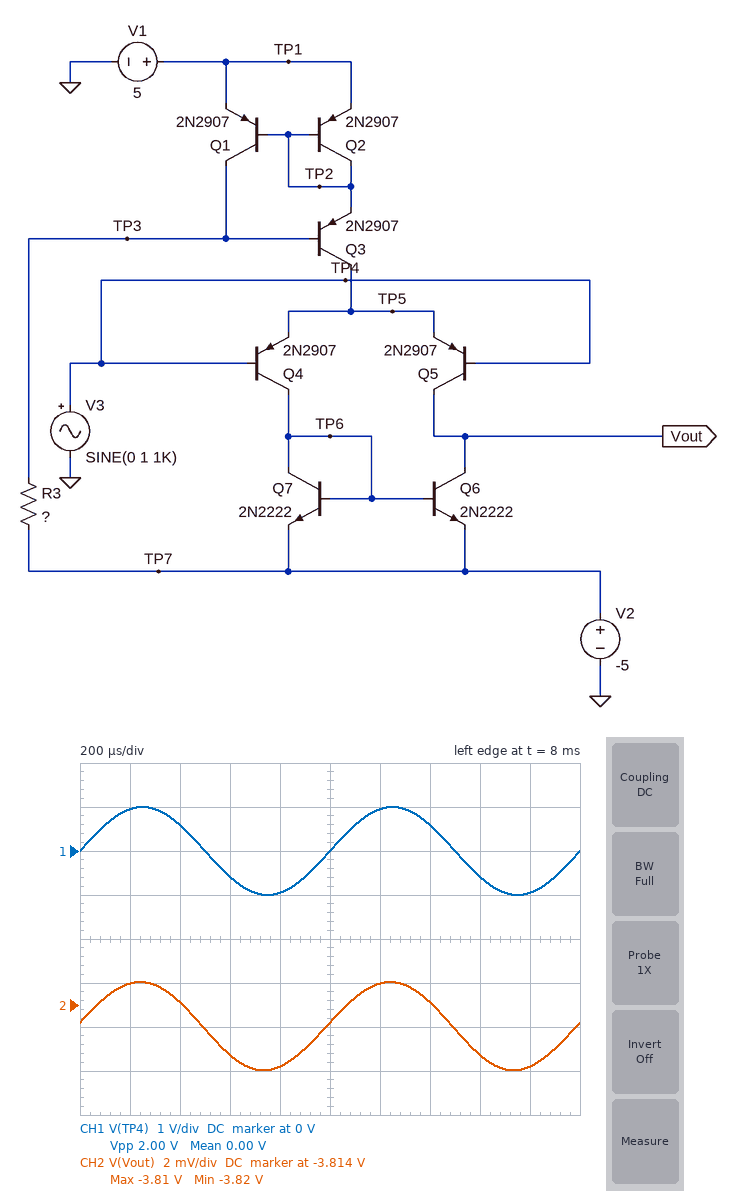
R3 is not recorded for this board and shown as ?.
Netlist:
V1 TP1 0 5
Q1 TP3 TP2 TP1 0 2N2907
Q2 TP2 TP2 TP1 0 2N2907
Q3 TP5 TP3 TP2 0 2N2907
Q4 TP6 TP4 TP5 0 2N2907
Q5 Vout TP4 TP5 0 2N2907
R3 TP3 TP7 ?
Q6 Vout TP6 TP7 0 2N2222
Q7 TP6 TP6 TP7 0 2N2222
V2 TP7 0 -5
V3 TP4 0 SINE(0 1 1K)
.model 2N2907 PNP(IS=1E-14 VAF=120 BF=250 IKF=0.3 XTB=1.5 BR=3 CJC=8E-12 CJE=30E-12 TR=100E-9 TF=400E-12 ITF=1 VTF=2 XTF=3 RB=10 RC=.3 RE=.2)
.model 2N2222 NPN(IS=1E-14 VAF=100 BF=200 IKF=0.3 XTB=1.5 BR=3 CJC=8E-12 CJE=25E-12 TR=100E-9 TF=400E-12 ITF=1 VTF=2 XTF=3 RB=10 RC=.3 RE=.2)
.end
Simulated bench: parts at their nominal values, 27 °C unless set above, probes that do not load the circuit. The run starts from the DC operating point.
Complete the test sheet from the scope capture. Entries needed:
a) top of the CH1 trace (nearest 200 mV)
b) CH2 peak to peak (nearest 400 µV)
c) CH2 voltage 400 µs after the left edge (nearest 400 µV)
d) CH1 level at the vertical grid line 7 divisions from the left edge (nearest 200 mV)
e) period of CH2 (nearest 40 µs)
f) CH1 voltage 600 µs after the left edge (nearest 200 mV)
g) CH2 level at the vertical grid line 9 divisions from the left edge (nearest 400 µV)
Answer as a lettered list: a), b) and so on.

a) 1.0 V
b) 4.0 mV
c) -3.8140 V
d) 600 mV
e) 1.00 ms
f) -600 mV
g) -3.8168 V
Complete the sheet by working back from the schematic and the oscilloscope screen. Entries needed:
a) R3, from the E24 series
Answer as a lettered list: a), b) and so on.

a) 11 kΩ
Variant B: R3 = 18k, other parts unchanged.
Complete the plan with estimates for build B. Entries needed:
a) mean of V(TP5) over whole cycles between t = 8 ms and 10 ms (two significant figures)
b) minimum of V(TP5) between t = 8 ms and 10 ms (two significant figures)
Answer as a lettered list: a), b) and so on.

a) 620 mV
b) -380 mV
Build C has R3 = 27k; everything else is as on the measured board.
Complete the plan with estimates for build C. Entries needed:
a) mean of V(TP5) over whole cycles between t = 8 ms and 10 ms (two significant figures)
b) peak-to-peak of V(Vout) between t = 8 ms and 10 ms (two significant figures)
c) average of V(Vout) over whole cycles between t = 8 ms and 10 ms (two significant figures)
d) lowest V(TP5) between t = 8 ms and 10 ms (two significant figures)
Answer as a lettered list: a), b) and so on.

a) 610 mV
b) 4.1 mV
c) -3.8 V
d) -390 mV
